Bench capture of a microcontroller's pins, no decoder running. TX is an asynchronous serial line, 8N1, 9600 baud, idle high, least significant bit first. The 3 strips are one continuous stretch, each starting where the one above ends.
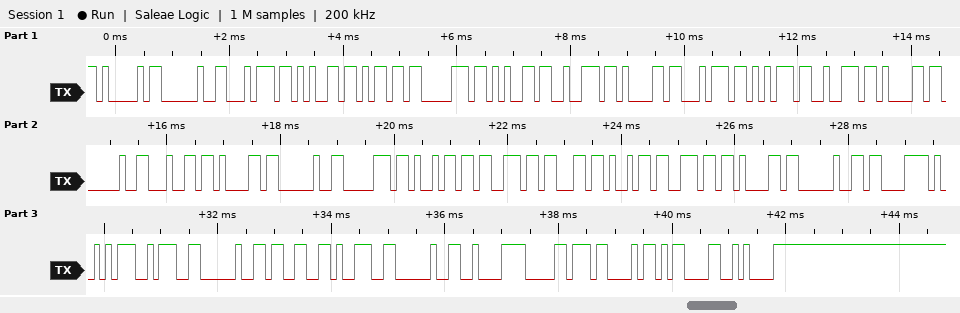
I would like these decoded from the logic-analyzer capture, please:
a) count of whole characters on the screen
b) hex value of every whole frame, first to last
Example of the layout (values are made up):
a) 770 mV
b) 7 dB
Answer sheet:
a) 37
b) 41 20 74 65 6D 70 65 72 61 74 75 72 61 20 64 61 20 70 69 73 63 69 6E 61 20 C3 A9 3A 20 33 39 20 C2 B0 43 0D 0A
